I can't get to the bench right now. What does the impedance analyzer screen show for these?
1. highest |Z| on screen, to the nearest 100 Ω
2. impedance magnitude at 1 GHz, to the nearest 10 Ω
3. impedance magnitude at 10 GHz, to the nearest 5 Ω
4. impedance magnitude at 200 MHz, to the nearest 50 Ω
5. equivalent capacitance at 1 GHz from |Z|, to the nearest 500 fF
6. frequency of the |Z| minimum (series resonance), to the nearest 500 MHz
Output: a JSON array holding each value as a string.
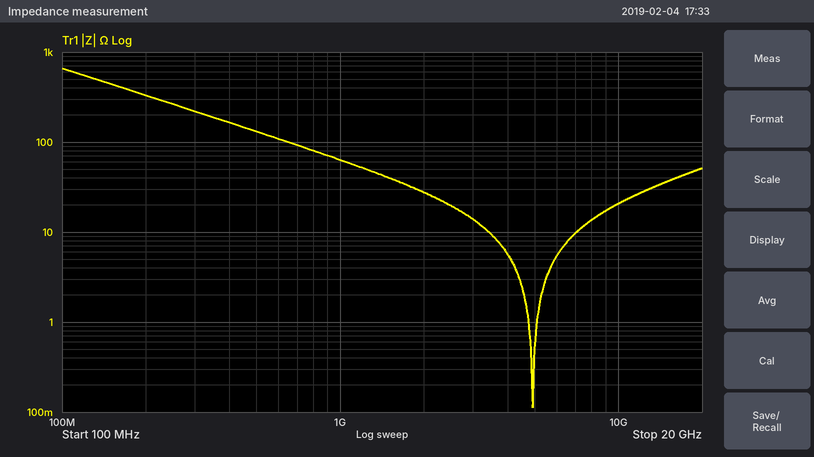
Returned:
["700 Ω", "60 Ω", "20 Ω", "350 Ω", "2.5 pF", "5.0 GHz"]
